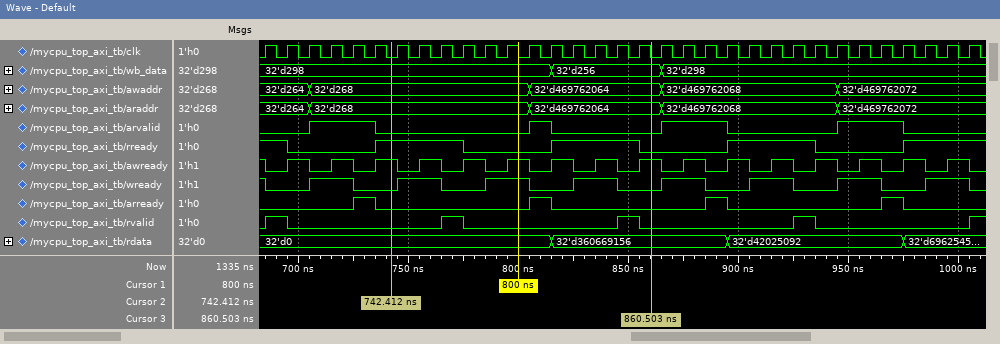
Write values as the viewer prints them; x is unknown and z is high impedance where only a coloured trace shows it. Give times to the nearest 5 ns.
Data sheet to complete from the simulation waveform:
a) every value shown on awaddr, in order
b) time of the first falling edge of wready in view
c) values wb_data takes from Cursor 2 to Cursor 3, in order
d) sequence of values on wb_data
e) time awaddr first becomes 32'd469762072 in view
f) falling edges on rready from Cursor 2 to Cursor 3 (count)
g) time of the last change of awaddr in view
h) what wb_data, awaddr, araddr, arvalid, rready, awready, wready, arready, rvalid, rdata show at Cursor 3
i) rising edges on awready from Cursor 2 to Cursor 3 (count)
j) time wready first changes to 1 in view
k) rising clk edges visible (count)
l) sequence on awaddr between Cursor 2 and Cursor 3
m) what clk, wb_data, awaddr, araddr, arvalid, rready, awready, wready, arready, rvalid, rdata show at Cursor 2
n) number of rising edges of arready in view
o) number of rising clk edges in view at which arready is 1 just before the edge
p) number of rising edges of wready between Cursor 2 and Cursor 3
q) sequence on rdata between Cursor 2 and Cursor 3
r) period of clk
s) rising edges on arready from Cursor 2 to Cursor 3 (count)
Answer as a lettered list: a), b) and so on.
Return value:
a) 32'd264, 32'd268, 32'd469762064, 32'd469762068, 32'd469762072
b) 685 ns
c) 32'd298, 32'd256
d) 32'd298, 32'd256, 32'd298
e) 945 ns
f) 2
g) 945 ns
h) wb_data=32'd256, awaddr=32'd469762064, araddr=32'd469762064, arvalid=0, rready=0, awready=1, wready=0, arready=0, rvalid=0, rdata=32'd360669156
i) 6
j) 705 ns
k) 33
l) 32'd268, 32'd469762064
m) clk=0, wb_data=32'd298, awaddr=32'd268, araddr=32'd268, arvalid=0, rready=1, awready=1, wready=0, arready=0, rvalid=0, rdata=32'd0
n) 4
o) 4
p) 3
q) 32'd0, 32'd360669156
r) 10 ns
s) 1
